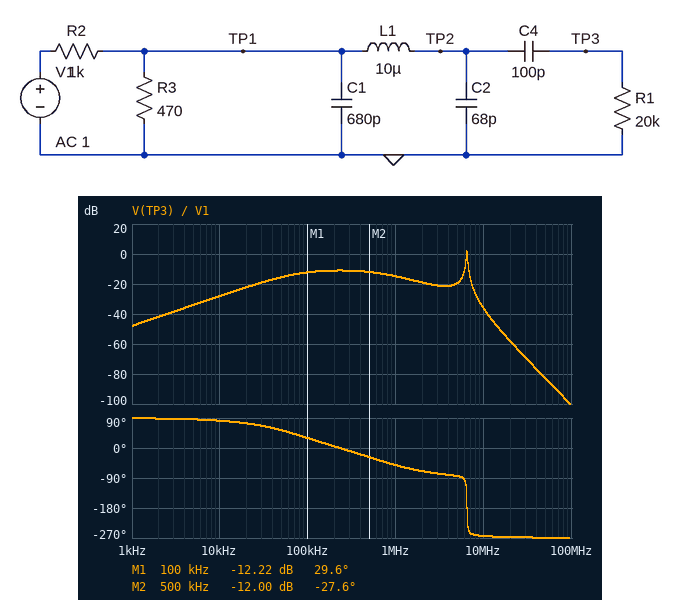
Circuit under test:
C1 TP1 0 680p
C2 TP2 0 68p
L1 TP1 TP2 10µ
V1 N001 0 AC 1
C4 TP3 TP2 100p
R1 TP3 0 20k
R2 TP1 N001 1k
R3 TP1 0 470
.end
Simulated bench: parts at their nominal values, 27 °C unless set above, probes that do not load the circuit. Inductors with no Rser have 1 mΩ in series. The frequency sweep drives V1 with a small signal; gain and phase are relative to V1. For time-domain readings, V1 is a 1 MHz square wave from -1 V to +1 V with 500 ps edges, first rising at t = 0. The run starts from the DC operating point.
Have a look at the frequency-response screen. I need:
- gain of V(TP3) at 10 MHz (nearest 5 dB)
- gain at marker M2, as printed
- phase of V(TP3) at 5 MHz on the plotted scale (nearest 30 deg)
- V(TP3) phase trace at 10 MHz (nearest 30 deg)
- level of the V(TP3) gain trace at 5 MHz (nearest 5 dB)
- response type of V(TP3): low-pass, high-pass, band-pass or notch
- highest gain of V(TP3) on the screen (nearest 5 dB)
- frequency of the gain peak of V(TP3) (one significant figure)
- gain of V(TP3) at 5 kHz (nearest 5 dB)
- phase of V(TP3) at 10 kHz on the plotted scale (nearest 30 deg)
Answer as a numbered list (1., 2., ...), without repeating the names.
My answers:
1. -35 dB
2. -12.00 dB
3. -90 deg
4. -270 deg
5. -20 dB
6. band-pass
7. 0 dB
8. 6 MHz
9. -35 dB
10. 90 deg
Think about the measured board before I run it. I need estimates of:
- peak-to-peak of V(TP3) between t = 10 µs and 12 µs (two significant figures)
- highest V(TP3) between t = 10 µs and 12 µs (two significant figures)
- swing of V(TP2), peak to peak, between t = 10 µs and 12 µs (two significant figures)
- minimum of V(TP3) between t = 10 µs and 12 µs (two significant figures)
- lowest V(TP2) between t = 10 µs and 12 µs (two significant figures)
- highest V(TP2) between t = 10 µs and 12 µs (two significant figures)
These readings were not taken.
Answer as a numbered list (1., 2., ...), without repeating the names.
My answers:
1. 520 mV
2. 260 mV
3. 530 mV
4. -260 mV
5. -270 mV
6. 270 mV
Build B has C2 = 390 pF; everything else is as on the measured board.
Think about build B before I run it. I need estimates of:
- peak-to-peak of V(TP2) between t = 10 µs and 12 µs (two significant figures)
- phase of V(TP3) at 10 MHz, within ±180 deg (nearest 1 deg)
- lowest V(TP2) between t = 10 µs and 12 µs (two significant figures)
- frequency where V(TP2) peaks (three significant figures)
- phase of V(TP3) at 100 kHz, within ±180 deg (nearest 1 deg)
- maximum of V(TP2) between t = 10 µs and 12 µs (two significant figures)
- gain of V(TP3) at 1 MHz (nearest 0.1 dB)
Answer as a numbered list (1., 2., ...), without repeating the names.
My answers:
1. 630 mV
2. 95 deg
3. -310 mV
4. 3.17 MHz
5. 26 deg
6. 310 mV
7. -16.5 dB
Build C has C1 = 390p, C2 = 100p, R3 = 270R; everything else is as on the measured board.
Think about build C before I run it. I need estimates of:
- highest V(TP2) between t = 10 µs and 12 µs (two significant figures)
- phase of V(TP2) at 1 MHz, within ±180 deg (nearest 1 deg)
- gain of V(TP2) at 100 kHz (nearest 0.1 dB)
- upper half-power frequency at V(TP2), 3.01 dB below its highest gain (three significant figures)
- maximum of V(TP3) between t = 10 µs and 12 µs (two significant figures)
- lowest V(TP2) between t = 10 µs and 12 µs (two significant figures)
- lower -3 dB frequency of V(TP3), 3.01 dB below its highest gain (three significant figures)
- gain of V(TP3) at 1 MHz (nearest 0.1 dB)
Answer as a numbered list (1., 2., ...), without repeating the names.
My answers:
1. 260 mV
2. -33 deg
3. -13.5 dB
4. 5.78 MHz
5. 260 mV
6. -260 mV
7. 5.35 MHz
8. -14.8 dB
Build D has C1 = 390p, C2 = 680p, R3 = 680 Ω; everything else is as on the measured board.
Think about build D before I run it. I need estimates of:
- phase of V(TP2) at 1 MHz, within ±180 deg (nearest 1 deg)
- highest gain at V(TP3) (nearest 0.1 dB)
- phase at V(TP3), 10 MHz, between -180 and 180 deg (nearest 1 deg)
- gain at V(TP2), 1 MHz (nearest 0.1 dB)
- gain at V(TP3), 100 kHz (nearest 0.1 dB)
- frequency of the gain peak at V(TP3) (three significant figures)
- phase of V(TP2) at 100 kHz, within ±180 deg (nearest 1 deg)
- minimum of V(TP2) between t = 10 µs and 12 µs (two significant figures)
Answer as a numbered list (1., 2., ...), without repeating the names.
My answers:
1. -73 deg
2. -9.6 dB
3. 97 deg
4. -16.1 dB
5. -10.4 dB
6. 175 kHz
7. -16 deg
8. -270 mV
